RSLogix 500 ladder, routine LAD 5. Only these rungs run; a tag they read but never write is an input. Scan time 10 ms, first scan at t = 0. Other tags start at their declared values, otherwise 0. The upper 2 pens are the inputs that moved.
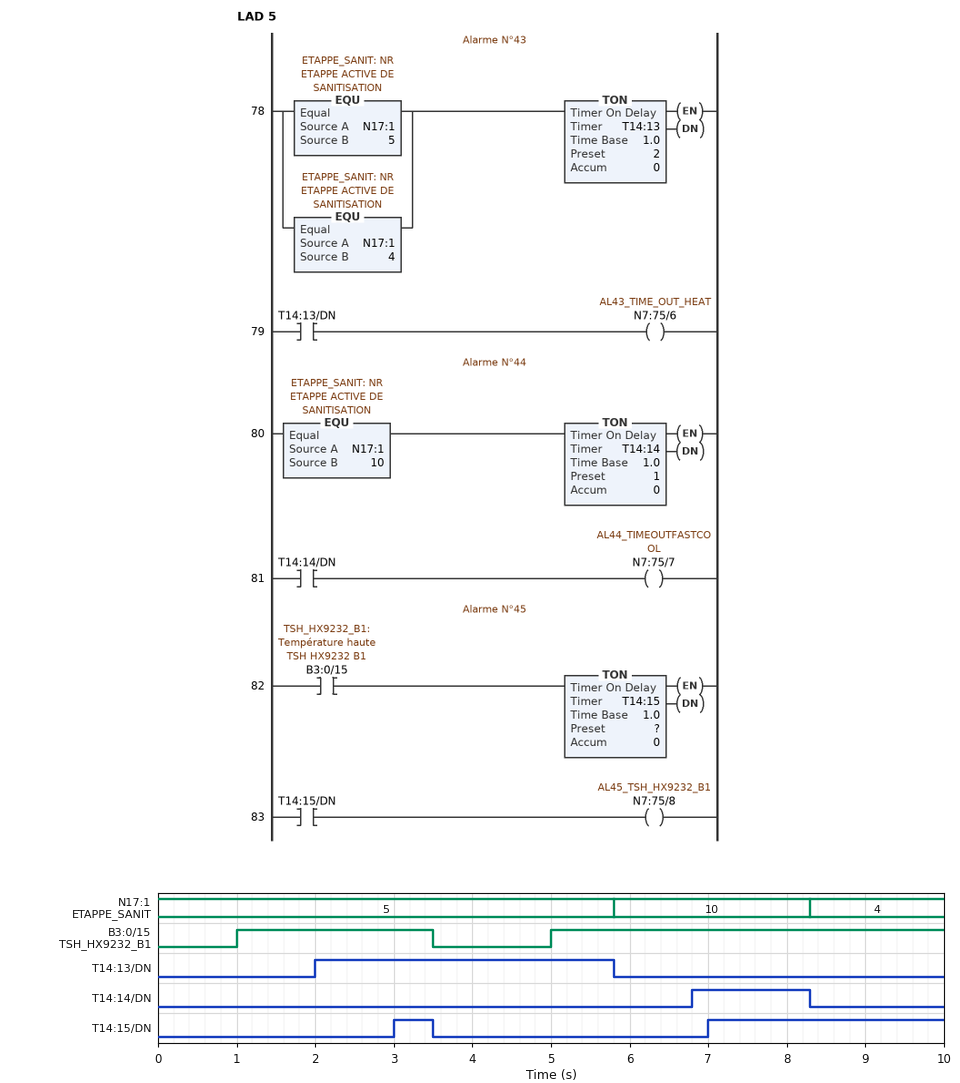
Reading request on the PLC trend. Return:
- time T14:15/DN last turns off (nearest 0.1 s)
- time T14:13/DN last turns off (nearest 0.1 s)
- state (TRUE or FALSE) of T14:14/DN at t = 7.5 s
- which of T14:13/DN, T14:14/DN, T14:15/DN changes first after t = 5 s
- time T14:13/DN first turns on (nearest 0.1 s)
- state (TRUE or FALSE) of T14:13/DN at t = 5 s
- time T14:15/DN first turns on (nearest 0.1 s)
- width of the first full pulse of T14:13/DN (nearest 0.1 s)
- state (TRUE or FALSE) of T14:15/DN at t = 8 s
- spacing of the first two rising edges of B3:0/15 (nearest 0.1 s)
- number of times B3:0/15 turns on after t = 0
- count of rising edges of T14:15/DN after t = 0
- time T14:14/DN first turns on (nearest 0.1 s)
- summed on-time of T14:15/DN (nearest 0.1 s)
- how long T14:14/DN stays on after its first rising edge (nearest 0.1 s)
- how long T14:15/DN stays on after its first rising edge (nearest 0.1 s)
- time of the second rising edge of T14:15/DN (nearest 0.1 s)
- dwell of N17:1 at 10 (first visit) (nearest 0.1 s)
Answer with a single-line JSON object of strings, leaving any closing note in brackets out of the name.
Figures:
{"time T14:15/DN last turns off": "3.5 s", "time T14:13/DN last turns off": "5.8 s", "state (TRUE or FALSE) of T14:14/DN at t = 7.5 s": "TRUE", "which of T14:13/DN, T14:14/DN, T14:15/DN changes first after t = 5 s": "T14:13/DN", "time T14:13/DN first turns on": "2.0 s", "state (TRUE or FALSE) of T14:13/DN at t = 5 s": "TRUE", "time T14:15/DN first turns on": "3.0 s", "width of the first full pulse of T14:13/DN": "3.8 s", "state (TRUE or FALSE) of T14:15/DN at t = 8 s": "TRUE", "spacing of the first two rising edges of B3:0/15": "4.0 s", "number of times B3:0/15 turns on after t = 0": "2", "count of rising edges of T14:15/DN after t = 0": "2", "time T14:14/DN first turns on": "6.8 s", "summed on-time of T14:15/DN": "3.5 s", "how long T14:14/DN stays on after its first rising edge": "1.5 s", "how long T14:15/DN stays on after its first rising edge": "0.5 s", "time of the second rising edge of T14:15/DN": "7.0 s", "dwell of N17:1 at 10 (first visit)": "2.5 s"}
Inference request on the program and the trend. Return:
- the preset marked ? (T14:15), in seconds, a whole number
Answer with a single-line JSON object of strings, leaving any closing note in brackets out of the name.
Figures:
{"the preset marked ? (T14:15), in seconds, a whole number": "2 s"}
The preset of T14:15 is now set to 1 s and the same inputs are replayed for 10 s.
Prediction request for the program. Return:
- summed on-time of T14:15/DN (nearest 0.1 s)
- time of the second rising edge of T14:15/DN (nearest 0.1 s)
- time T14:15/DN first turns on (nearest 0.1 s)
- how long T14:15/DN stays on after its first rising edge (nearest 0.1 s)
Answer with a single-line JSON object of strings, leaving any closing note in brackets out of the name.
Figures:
{"summed on-time of T14:15/DN": "5.5 s", "time of the second rising edge of T14:15/DN": "6.0 s", "time T14:15/DN first turns on": "2.0 s", "how long T14:15/DN stays on after its first rising edge": "1.5 s"}
